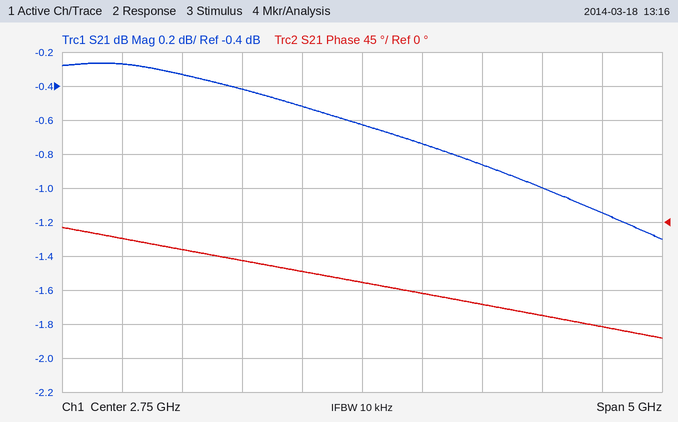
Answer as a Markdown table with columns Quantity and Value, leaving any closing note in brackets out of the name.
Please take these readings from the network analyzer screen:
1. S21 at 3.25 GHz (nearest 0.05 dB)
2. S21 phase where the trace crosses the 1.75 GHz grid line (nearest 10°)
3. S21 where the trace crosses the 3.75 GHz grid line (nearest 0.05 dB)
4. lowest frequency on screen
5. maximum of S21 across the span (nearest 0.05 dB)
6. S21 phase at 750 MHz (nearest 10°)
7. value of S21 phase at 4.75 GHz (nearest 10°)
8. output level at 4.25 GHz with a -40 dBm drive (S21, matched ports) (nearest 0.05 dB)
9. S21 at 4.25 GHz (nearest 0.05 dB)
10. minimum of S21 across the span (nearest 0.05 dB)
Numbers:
| Quantity | Value |
|---|---|
| S21 at 3.25 GHz | -0.75 dB |
| S21 phase where the trace crosses the 1.75 GHz grid line | -50° |
| S21 where the trace crosses the 3.75 GHz grid line | -0.85 dB |
| lowest frequency on screen | 250 MHz |
| maximum of S21 across the span | -0.25 dB |
| S21 phase at 750 MHz | -20° |
| value of S21 phase at 4.75 GHz | -140° |
| output level at 4.25 GHz with a -40 dBm drive (S21, matched ports) | -41.00 dBm |
| S21 at 4.25 GHz | -1.00 dB |
| minimum of S21 across the span | -1.30 dB |
